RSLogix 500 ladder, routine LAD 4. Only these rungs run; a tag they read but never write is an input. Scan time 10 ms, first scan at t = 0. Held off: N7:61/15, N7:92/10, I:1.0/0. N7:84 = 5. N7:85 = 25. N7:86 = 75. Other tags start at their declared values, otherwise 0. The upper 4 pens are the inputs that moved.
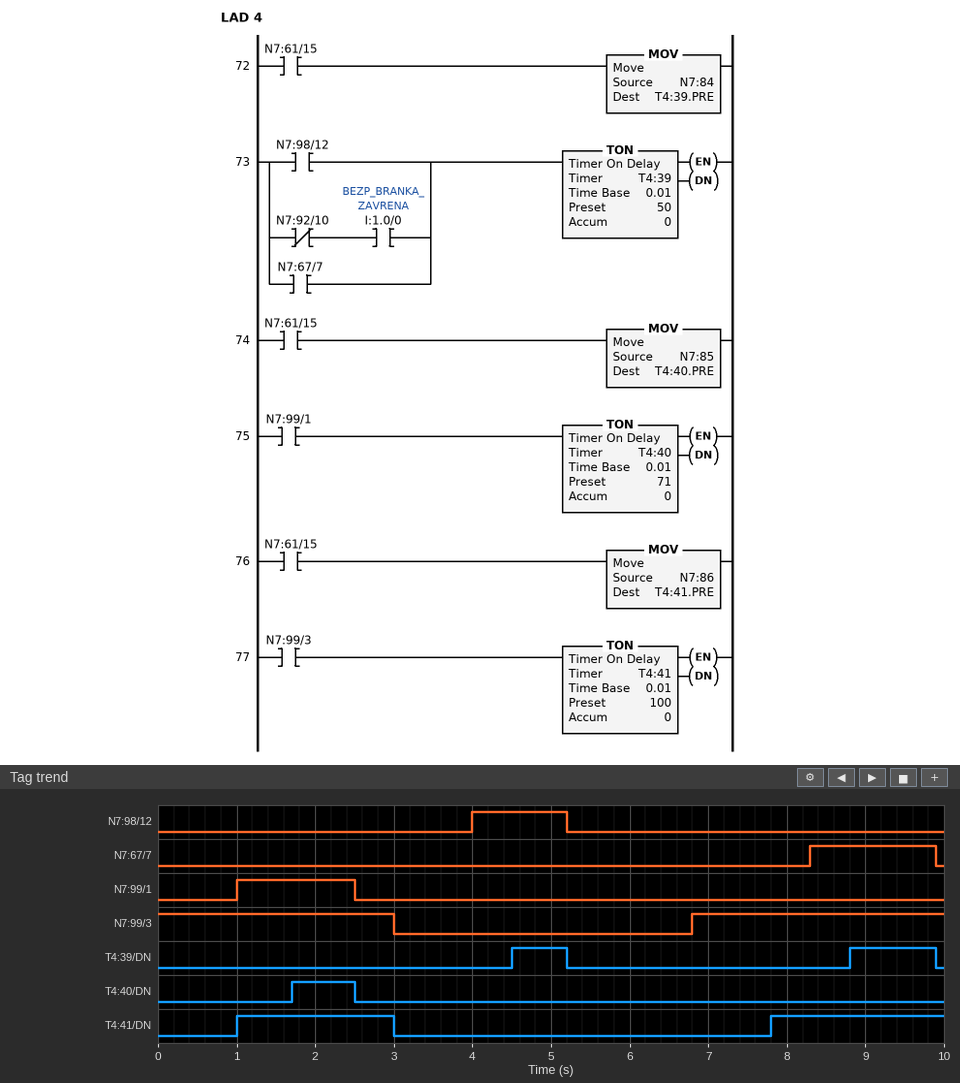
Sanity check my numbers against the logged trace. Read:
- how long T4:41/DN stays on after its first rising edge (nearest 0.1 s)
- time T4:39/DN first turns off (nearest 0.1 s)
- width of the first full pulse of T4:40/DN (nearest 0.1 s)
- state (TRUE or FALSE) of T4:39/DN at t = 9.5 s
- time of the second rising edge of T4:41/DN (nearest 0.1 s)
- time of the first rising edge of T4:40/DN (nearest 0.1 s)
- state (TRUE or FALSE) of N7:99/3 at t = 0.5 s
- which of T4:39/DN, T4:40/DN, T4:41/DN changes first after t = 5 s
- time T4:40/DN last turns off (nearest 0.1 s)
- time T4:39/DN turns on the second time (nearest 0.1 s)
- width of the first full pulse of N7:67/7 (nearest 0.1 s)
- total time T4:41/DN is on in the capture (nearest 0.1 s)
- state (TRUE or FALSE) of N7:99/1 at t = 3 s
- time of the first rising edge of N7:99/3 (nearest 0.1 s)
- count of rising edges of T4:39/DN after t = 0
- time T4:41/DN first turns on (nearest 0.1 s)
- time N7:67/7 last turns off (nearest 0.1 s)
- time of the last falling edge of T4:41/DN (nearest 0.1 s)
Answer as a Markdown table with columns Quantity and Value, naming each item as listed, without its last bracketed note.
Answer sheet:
| Quantity | Value |
|---|---|
| how long T4:41/DN stays on after its first rising edge | 2.0 s |
| time T4:39/DN first turns off | 5.2 s |
| width of the first full pulse of T4:40/DN | 0.8 s |
| state (TRUE or FALSE) of T4:39/DN at t = 9.5 s | TRUE |
| time of the second rising edge of T4:41/DN | 7.8 s |
| time of the first rising edge of T4:40/DN | 1.7 s |
| state (TRUE or FALSE) of N7:99/3 at t = 0.5 s | TRUE |
| which of T4:39/DN, T4:40/DN, T4:41/DN changes first after t = 5 s | T4:39/DN |
| time T4:40/DN last turns off | 2.5 s |
| time T4:39/DN turns on the second time | 8.8 s |
| width of the first full pulse of N7:67/7 | 1.6 s |
| total time T4:41/DN is on in the capture | 4.2 s |
| state (TRUE or FALSE) of N7:99/1 at t = 3 s | FALSE |
| time of the first rising edge of N7:99/3 | 6.8 s |
| count of rising edges of T4:39/DN after t = 0 | 2 |
| time T4:41/DN first turns on | 1.0 s |
| time N7:67/7 last turns off | 9.9 s |
| time of the last falling edge of T4:41/DN | 3.0 s |
